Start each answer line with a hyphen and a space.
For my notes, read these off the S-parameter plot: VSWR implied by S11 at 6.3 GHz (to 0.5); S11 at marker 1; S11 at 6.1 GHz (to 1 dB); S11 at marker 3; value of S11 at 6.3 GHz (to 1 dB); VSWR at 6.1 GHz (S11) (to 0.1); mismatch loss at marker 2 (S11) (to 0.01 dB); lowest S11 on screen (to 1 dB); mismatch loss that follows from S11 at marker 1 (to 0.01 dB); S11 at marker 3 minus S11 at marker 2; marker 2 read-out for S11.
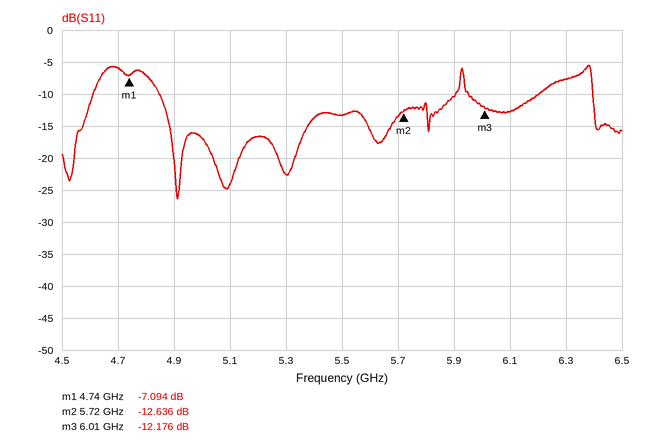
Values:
- 2.5
- -7.094 dB
- -13 dB
- -12.176 dB
- -8 dB
- 1.6
- 0.24 dB
- -26 dB
- 0.94 dB
- 0.460 dB
- -12.636 dB
